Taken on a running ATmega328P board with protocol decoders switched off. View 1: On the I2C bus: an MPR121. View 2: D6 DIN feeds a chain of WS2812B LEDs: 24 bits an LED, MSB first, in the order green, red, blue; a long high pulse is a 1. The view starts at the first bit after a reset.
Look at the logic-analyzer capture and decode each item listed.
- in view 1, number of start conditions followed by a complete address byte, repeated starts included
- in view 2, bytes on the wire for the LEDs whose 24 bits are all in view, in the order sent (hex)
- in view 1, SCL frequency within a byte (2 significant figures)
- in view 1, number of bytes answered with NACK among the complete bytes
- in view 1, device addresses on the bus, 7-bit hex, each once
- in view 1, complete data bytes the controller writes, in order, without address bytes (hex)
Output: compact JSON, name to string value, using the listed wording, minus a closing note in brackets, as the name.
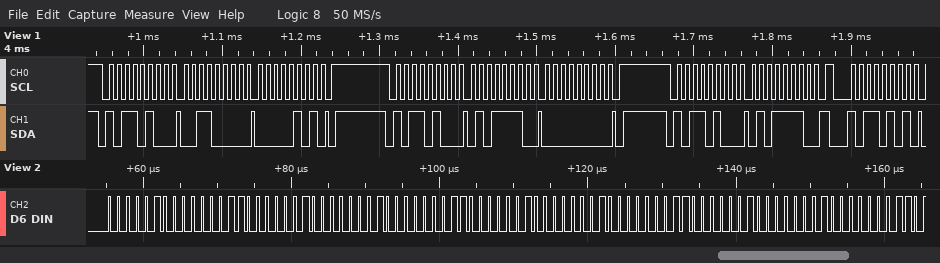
{"in view 1, number of start conditions followed by a complete address byte, repeated starts included": "4", "in view 2, bytes on the wire for the LEDs whose 24 bits are all in view, in the order sent": "04 06 04 04 06 04 04 06 04", "in view 1, SCL frequency within a byte": "100 kHz", "in view 1, number of bytes answered with NACK among the complete bytes": "0", "in view 1, device addresses on the bus, 7-bit hex, each once": "0x5A", "in view 1, complete data bytes the controller writes, in order, without address bytes": "30 05 5E 00 5E"}
